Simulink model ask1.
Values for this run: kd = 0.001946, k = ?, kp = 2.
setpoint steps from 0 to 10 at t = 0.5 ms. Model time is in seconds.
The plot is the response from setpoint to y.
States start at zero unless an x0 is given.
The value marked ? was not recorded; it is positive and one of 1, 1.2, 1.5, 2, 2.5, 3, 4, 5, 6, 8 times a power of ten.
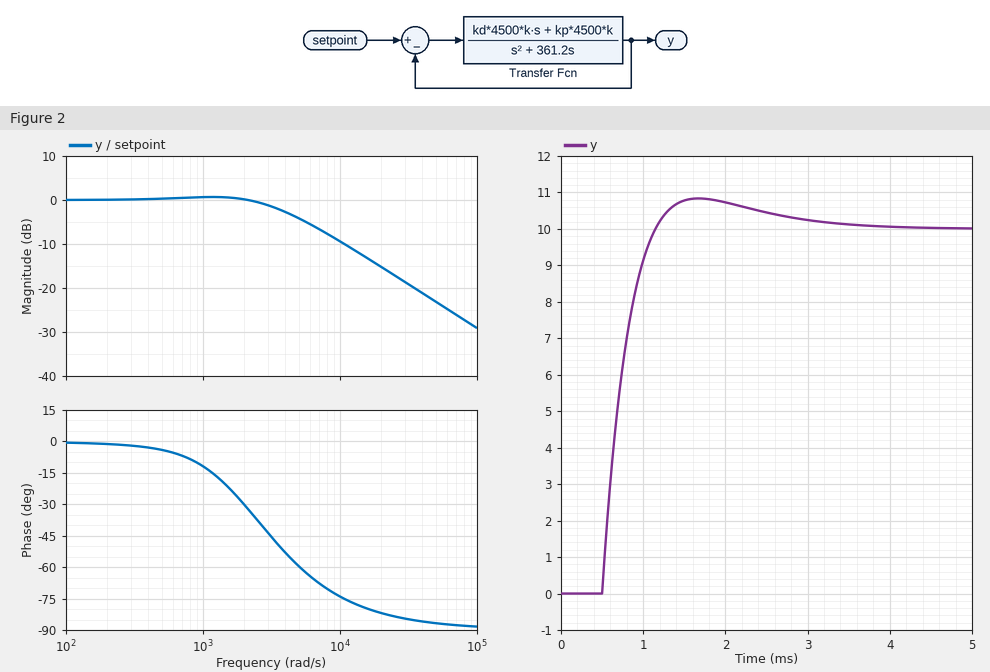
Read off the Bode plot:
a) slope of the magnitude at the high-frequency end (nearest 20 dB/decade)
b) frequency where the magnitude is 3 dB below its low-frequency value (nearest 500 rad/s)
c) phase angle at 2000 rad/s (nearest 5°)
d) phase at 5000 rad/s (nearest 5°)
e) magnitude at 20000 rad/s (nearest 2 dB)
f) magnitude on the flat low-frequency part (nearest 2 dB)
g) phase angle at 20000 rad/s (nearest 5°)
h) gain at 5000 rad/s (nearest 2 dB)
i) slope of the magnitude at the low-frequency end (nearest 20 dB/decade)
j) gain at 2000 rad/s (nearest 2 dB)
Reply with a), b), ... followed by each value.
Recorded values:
a) -20 dB/decade
b) 4000 rad/s
c) -30°
d) -60°
e) -16 dB
f) 0 dB
g) -80°
h) -4 dB
i) 0 dB/decade
j) 0 dB
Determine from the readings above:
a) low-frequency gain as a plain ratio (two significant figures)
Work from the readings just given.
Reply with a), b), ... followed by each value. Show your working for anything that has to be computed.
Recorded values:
a) 10^(0 / 20) = 1.0
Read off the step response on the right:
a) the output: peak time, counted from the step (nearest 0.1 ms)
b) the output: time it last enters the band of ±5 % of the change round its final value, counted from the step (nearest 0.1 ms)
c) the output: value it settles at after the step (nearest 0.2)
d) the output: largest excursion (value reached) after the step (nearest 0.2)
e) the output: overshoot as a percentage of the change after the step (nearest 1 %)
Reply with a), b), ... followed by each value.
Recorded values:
a) 1.2 ms
b) 1.9 ms
c) 10.0
d) 10.8
e) 8 %
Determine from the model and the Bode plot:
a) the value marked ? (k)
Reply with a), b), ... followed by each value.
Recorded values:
a) 400
